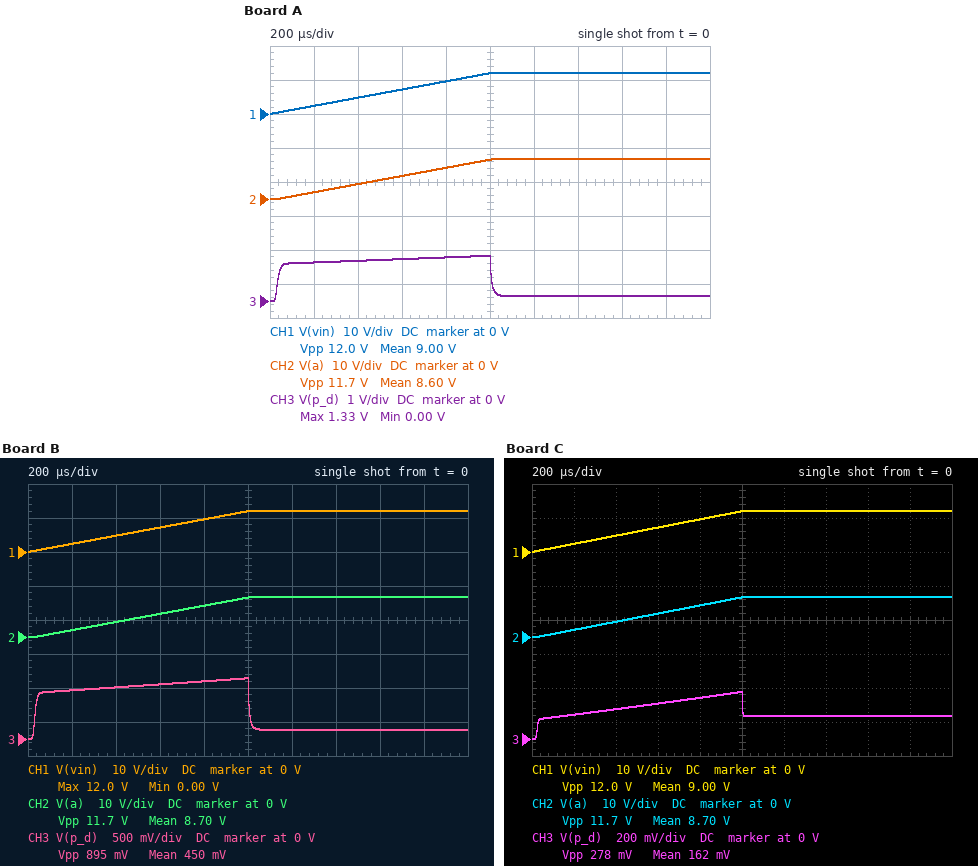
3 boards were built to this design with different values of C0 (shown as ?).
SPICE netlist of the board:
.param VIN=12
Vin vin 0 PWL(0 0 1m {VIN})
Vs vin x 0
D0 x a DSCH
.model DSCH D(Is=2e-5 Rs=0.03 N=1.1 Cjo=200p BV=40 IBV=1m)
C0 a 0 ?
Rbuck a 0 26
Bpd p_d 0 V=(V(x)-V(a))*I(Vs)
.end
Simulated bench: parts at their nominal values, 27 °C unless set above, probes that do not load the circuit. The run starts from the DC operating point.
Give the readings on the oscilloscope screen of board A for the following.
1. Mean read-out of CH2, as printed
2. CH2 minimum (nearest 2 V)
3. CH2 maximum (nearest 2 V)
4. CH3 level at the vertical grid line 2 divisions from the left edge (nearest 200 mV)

8.60 V
0 V
12 V
1.2 V
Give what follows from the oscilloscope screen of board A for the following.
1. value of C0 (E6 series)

220 µF
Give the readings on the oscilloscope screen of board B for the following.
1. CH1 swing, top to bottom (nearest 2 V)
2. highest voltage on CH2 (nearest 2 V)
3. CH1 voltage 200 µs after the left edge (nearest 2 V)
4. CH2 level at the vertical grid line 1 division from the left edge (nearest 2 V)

12 V
12 V
2 V
2 V
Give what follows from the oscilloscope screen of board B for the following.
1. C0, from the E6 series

150 µF
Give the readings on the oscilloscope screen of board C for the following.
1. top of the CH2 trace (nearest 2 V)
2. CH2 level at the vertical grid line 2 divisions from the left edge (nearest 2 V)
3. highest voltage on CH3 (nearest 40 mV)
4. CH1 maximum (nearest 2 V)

12 V
4 V
280 mV
12 V
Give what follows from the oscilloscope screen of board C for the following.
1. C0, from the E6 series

33 µF
